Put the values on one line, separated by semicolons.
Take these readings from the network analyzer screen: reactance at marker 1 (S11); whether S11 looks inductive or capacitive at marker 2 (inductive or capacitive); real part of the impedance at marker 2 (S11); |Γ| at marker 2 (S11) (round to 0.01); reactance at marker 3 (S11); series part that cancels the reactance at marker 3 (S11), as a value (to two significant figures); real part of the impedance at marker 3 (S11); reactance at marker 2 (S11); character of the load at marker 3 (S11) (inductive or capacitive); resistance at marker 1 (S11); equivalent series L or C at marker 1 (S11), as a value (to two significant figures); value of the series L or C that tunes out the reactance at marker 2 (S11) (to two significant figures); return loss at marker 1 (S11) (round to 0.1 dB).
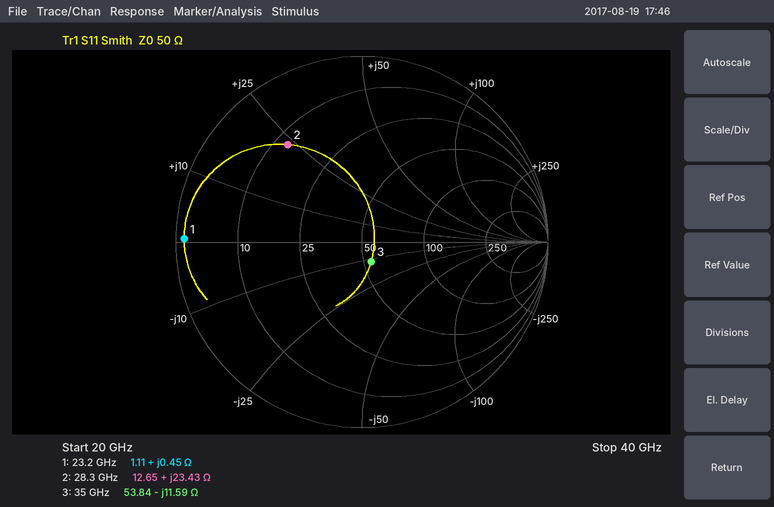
+0.45 Ω; inductive; 12.65 Ω; 0.66; -11.59 Ω; 53 pH; 53.84 Ω; +23.43 Ω; capacitive; 1.11 Ω; 3.1 pH; 240 fF; 0.4 dB
